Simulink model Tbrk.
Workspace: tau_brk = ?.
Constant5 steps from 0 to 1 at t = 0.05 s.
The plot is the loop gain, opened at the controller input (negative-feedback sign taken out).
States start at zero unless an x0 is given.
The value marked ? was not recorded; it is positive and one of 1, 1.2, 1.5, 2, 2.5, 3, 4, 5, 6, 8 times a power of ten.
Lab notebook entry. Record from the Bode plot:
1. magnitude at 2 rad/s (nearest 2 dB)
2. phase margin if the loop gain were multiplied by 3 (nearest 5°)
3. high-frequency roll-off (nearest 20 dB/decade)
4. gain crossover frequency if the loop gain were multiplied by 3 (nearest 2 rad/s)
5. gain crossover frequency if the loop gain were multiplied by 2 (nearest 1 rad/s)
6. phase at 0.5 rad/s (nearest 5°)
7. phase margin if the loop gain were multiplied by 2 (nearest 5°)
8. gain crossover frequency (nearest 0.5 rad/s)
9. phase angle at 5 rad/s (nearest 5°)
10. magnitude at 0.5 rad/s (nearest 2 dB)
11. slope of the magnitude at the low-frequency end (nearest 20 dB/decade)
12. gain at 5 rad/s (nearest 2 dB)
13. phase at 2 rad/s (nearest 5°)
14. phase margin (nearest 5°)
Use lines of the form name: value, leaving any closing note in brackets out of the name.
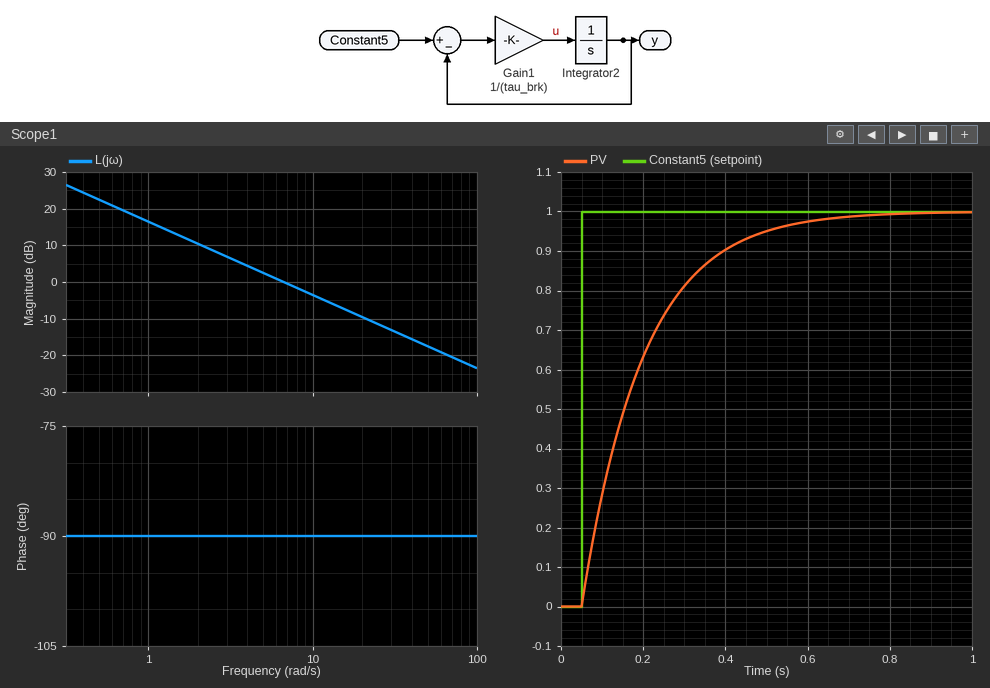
magnitude at 2 rad/s: 10 dB
phase margin if the loop gain were multiplied by 3: 90°
high-frequency roll-off: -20 dB/decade
gain crossover frequency if the loop gain were multiplied by 3: 20 rad/s
gain crossover frequency if the loop gain were multiplied by 2: 13 rad/s
phase at 0.5 rad/s: -90°
phase margin if the loop gain were multiplied by 2: 90°
gain crossover frequency: 6.5 rad/s
phase angle at 5 rad/s: -90°
magnitude at 0.5 rad/s: 22 dB
slope of the magnitude at the low-frequency end: -20 dB/decade
gain at 5 rad/s: 2 dB
phase at 2 rad/s: -90°
phase margin: 90°
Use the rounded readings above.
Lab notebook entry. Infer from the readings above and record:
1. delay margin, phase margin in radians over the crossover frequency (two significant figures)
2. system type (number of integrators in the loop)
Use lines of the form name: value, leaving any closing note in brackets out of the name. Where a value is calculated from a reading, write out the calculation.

delay margin, phase margin in radians over the crossover frequency: 90 × π / 180 / 6.5 = 0.24 s
system type: 1
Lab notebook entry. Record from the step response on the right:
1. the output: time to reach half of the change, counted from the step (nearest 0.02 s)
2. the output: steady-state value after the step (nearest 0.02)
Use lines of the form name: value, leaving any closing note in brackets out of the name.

the output: time to reach half of the change, counted from the step: 0.10 s
the output: steady-state value after the step: 1.00
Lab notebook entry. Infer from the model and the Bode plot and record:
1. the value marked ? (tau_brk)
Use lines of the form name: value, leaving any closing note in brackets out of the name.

the value marked ?: 0.15
